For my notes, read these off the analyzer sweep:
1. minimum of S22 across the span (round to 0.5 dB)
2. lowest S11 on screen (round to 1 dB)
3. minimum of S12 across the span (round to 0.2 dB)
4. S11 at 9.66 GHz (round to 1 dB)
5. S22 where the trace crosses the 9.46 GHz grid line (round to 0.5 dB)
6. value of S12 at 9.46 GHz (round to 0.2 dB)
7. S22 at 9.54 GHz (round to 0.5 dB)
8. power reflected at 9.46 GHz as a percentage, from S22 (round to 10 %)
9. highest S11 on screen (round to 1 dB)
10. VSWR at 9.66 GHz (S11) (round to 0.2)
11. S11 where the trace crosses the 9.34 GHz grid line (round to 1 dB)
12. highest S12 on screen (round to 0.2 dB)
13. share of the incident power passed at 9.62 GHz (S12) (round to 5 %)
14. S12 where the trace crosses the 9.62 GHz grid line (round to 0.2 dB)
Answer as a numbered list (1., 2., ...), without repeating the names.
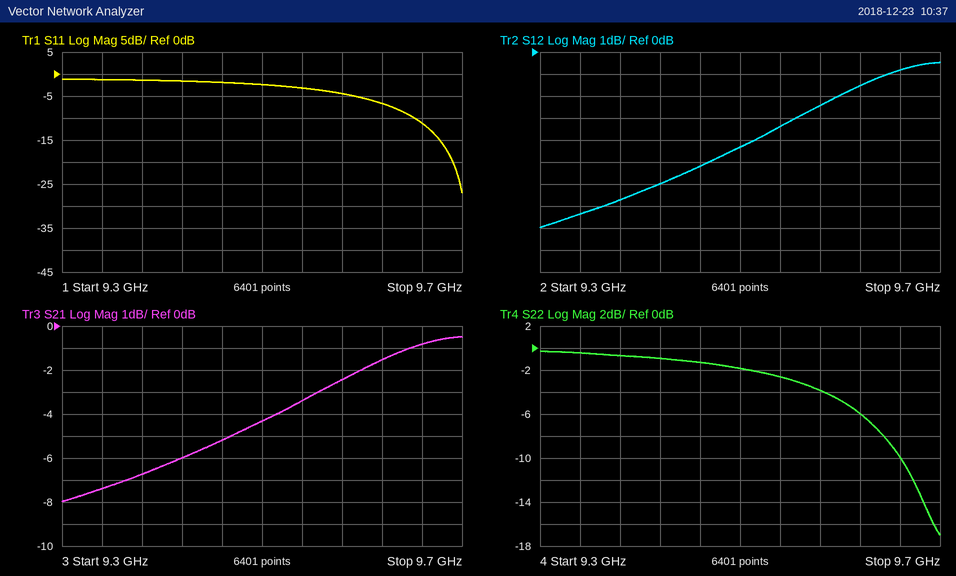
1. -17.0 dB
2. -27 dB
3. -8.0 dB
4. -11 dB
5. -1.5 dB
6. -5.2 dB
7. -2.5 dB
8. 70 %
9. -1 dB
10. 1.8
11. -1 dB
12. -0.4 dB
13. 70 %
14. -1.6 dB
